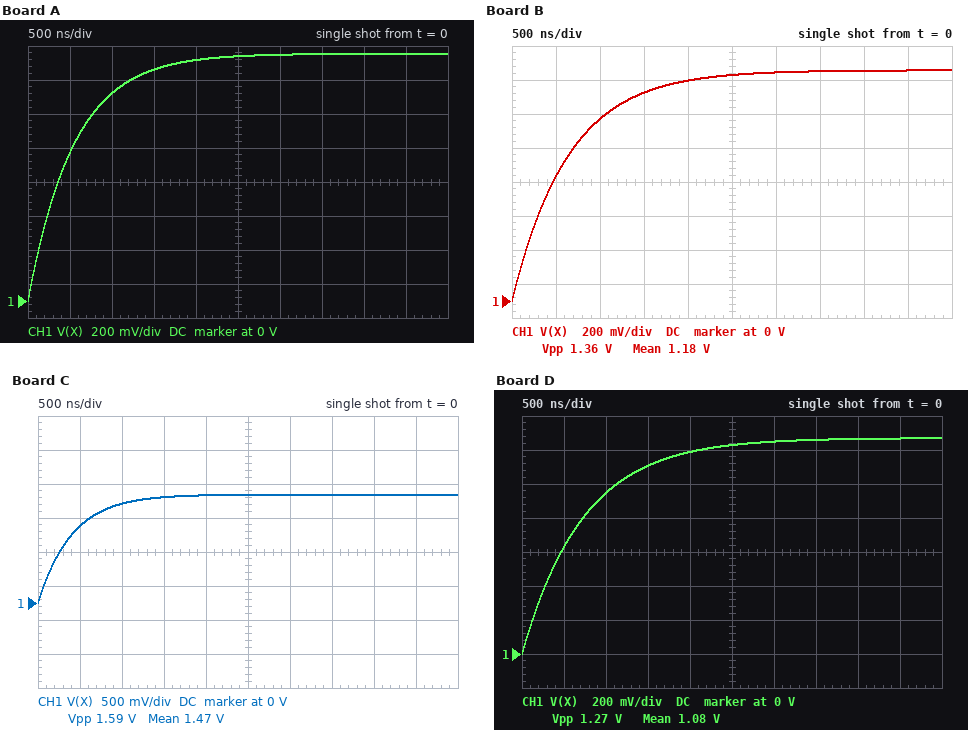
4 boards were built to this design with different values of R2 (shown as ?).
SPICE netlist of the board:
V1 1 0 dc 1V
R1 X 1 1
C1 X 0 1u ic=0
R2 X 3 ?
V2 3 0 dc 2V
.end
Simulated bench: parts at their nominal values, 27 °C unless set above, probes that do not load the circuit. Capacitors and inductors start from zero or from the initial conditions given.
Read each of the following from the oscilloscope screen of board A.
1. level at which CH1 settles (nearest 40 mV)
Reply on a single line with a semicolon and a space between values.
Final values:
1.44 V
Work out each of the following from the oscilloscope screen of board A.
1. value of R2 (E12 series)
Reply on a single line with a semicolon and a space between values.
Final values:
1.2 Ω
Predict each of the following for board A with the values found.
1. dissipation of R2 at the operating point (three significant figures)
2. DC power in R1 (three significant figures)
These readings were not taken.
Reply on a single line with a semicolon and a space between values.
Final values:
248 mW; 207 mW
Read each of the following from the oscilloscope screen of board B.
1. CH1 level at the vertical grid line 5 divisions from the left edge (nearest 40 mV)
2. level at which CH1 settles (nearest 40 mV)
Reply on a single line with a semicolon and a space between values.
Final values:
1.32 V; 1.36 V
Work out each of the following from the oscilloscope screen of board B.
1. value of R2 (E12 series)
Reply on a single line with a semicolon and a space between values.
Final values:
1.8 Ω
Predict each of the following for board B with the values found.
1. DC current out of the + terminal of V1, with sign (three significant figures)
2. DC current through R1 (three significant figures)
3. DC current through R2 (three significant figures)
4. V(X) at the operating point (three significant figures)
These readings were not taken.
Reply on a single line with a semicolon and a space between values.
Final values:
-357 mA; 357 mA; 357 mA; 1.36 V
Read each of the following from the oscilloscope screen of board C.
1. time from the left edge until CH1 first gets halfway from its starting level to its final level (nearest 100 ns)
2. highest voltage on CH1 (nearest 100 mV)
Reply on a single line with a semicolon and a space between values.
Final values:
300 ns; 1.6 V
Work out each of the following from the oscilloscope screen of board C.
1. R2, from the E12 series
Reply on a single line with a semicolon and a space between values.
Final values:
0.68 Ω
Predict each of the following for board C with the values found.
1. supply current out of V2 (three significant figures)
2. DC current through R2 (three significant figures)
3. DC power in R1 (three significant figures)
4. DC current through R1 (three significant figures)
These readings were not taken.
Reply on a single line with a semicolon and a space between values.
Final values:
595 mA; 595 mA; 354 mW; 595 mA
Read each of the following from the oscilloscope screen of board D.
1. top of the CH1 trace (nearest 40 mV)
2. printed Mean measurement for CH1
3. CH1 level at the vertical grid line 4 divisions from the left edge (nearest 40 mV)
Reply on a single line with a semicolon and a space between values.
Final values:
1.28 V; 1.08 V; 1.20 V
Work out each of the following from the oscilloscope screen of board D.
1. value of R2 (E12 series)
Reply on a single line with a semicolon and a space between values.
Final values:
2.7 Ω
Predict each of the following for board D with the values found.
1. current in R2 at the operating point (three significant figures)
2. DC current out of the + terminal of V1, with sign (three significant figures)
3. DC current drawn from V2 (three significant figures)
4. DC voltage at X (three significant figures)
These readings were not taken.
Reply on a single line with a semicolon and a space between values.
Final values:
270 mA; -270 mA; 270 mA; 1.27 V
